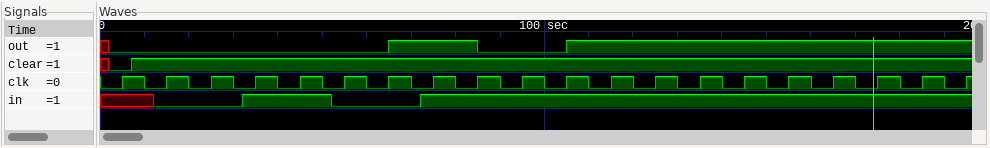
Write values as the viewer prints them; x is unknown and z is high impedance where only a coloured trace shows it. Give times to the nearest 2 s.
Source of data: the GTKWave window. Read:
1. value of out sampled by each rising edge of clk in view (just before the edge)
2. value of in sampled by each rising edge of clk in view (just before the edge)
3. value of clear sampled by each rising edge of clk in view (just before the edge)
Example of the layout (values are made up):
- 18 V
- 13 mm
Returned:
- 0 0 0 0 0 0 0 1 1 0 0 1 1 1 1 1 1 1 1 1
- x 0 0 1 1 0 0 1 1 1 1 1 1 1 1 1 1 1 1 1
- 0 1 1 1 1 1 1 1 1 1 1 1 1 1 1 1 1 1 1 1
